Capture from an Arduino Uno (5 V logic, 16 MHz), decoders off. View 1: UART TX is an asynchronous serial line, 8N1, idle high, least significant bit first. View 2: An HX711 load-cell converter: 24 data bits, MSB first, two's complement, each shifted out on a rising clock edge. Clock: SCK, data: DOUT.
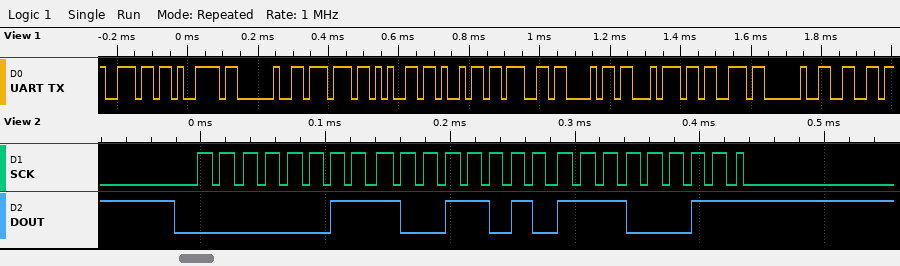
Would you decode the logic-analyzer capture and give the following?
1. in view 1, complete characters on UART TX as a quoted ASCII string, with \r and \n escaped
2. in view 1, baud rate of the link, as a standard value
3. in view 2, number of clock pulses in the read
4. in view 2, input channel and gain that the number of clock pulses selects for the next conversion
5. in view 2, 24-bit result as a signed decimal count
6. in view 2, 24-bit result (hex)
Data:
"ny weights f"
57600 baud
25
channel A, gain 128
236259
0x039AE3
